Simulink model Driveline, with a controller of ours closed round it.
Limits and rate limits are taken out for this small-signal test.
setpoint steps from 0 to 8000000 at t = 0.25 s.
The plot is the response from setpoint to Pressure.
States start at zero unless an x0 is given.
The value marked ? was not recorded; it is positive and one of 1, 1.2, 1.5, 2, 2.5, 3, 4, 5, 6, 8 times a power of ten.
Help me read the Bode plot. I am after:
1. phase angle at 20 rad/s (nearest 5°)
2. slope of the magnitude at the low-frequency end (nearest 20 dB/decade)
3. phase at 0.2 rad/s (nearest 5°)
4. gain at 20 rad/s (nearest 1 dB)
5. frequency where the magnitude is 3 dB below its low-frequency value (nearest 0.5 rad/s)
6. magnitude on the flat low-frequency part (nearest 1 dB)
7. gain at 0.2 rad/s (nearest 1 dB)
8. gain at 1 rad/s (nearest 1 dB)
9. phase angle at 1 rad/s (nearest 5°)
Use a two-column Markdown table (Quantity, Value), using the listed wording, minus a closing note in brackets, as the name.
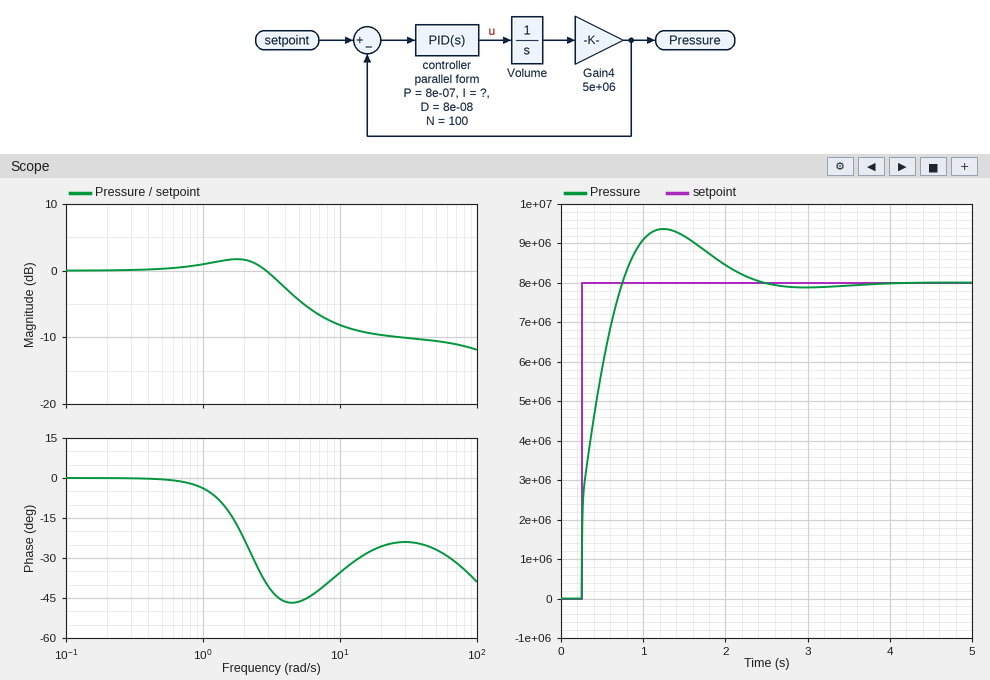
| Quantity | Value |
|---|---|
| phase angle at 20 rad/s | -25° |
| slope of the magnitude at the low-frequency end | 0 dB/decade |
| phase at 0.2 rad/s | 0° |
| gain at 20 rad/s | -10 dB |
| frequency where the magnitude is 3 dB below its low-frequency value | 4.0 rad/s |
| magnitude on the flat low-frequency part | 0 dB |
| gain at 0.2 rad/s | 0 dB |
| gain at 1 rad/s | 1 dB |
| phase angle at 1 rad/s | -5° |
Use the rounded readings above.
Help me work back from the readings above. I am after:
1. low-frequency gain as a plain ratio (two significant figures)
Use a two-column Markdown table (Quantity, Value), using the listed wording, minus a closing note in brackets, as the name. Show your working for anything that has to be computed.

| Quantity | Value |
|---|---|
| low-frequency gain as a plain ratio | 10^(0 / 20) = 1.0 |
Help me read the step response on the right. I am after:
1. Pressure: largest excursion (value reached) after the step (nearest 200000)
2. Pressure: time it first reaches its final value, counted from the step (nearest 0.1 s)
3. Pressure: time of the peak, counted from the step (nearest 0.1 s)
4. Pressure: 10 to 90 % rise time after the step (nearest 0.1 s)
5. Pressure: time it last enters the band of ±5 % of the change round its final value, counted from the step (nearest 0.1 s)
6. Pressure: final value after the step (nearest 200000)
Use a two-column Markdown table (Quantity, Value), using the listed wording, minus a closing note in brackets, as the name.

| Quantity | Value |
|---|---|
| Pressure: largest excursion (value reached) after the step | 9400000 |
| Pressure: time it first reaches its final value, counted from the step | 0.5 s |
| Pressure: time of the peak, counted from the step | 1.0 s |
| Pressure: 10 to 90 % rise time after the step | 0.4 s |
| Pressure: time it last enters the band of ±5 % of the change round its final value, counted from the step | 1.8 s |
| Pressure: final value after the step | 8000000 |
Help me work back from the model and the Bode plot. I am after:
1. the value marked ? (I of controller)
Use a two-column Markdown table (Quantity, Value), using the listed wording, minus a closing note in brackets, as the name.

| Quantity | Value |
|---|---|
| the value marked ? | 1.5e-06 |
